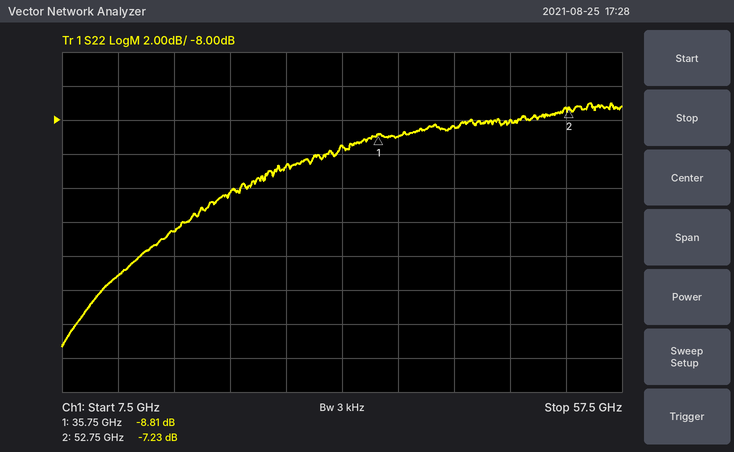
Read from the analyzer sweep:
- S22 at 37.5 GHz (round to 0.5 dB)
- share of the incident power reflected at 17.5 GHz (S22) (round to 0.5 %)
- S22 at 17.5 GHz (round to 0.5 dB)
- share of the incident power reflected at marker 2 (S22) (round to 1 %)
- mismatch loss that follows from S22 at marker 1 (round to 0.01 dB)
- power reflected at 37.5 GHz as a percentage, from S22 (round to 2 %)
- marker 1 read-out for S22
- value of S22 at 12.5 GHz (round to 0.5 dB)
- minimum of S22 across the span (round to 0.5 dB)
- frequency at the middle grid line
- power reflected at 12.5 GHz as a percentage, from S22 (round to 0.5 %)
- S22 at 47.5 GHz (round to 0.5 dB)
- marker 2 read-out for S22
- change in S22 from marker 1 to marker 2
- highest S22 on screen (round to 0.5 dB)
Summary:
-9.0 dB
3.5 %
-14.5 dB
19 %
0.61 dB
12 %
-8.81 dB
-17.0 dB
-21.5 dB
32.5 GHz
2.0 %
-8.0 dB
-7.23 dB
1.58 dB
-7.0 dB
